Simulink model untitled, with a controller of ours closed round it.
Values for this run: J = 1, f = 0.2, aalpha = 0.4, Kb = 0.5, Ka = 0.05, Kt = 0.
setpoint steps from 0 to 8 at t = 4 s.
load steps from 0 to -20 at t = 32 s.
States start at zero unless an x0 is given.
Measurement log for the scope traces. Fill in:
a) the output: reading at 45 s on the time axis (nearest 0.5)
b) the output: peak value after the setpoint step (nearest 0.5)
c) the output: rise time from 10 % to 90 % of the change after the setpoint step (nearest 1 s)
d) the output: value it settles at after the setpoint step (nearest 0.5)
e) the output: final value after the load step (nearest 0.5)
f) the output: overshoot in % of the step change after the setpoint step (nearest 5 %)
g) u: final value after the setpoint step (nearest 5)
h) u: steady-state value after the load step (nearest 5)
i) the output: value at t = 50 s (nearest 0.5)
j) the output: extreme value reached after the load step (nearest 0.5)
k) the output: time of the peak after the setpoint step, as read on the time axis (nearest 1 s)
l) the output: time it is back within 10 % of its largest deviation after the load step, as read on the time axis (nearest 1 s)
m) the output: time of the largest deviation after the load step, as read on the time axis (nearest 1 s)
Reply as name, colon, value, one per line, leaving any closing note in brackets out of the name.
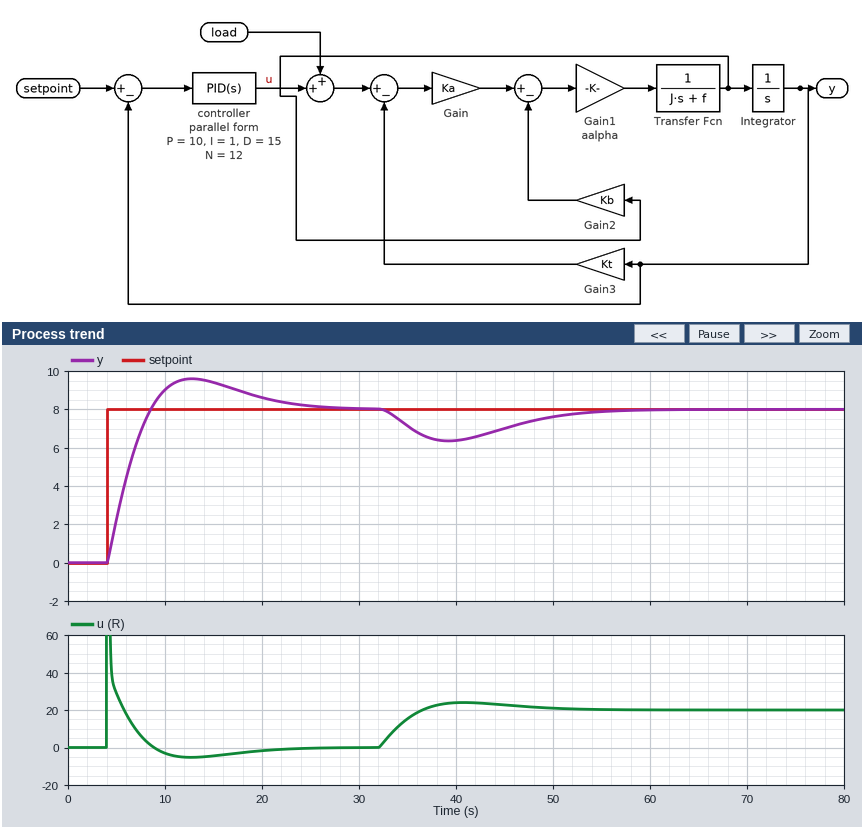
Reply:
the output: reading at 45 s on the time axis: 7.0
the output: peak value after the setpoint step: 9.5
the output: rise time from 10 % to 90 % of the change after the setpoint step: 3 s
the output: value it settles at after the setpoint step: 8.0
the output: final value after the load step: 8.0
the output: overshoot in % of the step change after the setpoint step: 20 %
u: final value after the setpoint step: 0
u: steady-state value after the load step: 20
the output: value at t = 50 s: 7.5
the output: extreme value reached after the load step: 6.5
the output: time of the peak after the setpoint step, as read on the time axis: 13 s
the output: time it is back within 10 % of its largest deviation after the load step, as read on the time axis: 54 s
the output: time of the largest deviation after the load step, as read on the time axis: 39 s
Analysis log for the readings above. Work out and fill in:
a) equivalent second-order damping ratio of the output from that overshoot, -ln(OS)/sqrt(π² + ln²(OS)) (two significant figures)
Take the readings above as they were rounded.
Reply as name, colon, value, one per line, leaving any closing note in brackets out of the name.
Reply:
equivalent second-order damping ratio of the output from that overshoot, -ln(OS)/sqrt(π² + ln²(OS)): 0.46
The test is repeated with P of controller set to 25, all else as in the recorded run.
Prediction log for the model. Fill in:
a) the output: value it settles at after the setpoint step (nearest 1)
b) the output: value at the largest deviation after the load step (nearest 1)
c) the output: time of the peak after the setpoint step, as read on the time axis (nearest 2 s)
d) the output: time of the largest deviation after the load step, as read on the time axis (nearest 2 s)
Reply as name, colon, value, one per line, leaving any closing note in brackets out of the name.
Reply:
the output: value it settles at after the setpoint step: 8
the output: value at the largest deviation after the load step: 7
the output: time of the peak after the setpoint step, as read on the time axis: 8 s
the output: time of the largest deviation after the load step, as read on the time axis: 36 s
